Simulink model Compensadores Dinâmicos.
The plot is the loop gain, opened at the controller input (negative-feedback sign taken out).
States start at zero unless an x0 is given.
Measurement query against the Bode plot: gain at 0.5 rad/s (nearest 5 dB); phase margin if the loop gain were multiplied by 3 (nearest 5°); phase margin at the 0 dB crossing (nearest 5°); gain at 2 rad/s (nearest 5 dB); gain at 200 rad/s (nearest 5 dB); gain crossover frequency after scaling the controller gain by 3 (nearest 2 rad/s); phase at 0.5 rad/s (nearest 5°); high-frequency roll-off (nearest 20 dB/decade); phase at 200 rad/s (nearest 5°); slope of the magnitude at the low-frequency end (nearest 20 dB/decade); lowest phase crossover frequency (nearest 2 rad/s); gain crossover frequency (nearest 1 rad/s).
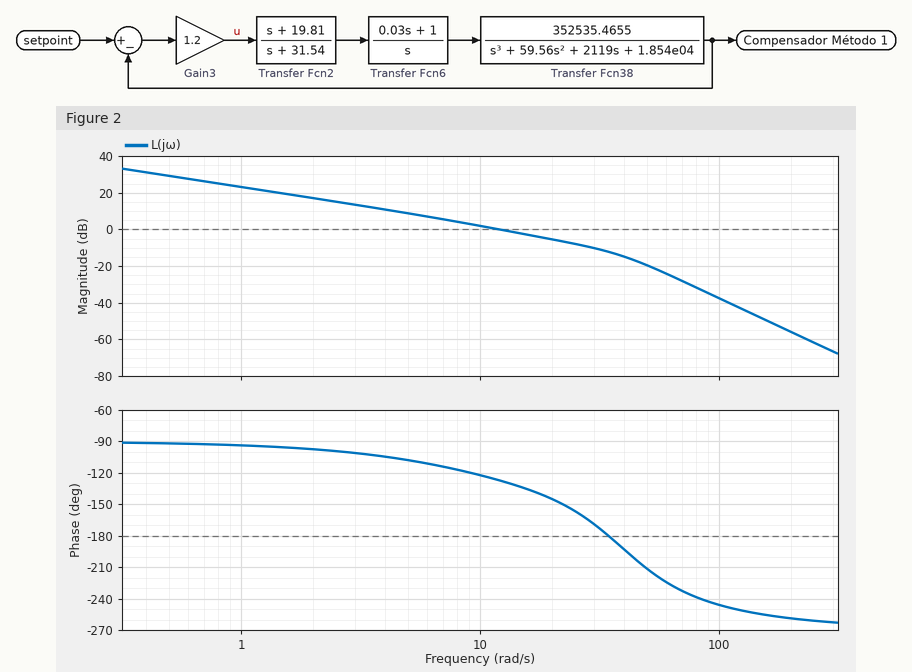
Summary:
30 dB
15°
55°
15 dB
-55 dB
28 rad/s
-90°
-60 dB/decade
-260°
-20 dB/decade
34 rad/s
12 rad/s
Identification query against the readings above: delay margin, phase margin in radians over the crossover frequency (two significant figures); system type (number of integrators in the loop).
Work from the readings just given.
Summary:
0.080 s
1
